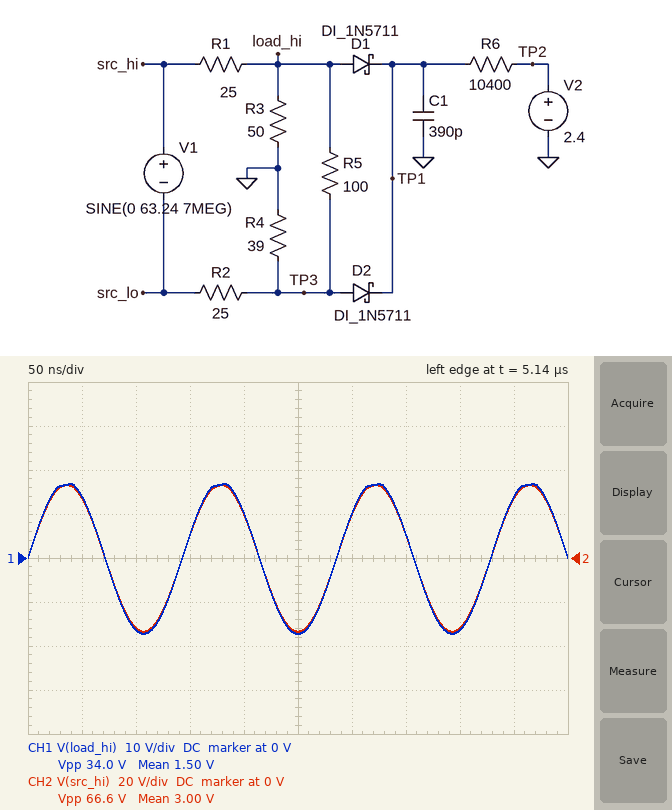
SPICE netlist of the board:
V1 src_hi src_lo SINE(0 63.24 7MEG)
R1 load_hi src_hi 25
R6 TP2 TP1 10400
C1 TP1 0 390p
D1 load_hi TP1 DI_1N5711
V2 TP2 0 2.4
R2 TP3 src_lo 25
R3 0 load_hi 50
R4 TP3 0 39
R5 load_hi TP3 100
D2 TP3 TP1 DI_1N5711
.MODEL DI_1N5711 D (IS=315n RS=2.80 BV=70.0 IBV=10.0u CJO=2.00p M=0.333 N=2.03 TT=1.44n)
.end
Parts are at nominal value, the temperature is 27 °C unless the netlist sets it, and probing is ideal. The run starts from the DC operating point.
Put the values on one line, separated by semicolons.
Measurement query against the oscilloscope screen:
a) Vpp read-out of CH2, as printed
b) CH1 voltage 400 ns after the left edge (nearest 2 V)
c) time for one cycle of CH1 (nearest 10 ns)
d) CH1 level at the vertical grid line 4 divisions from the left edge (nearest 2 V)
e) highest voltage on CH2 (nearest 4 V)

66.6 V; -16 V; 140 ns; 10 V; 32 V
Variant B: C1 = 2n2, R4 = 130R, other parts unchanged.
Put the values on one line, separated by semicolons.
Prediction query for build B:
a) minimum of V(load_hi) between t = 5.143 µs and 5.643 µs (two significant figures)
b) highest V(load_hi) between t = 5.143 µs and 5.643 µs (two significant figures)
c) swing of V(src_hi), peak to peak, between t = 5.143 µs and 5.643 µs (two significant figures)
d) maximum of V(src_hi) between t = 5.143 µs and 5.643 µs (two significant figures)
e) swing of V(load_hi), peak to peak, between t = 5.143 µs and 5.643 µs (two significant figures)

-11 V; 9.9 V; 49 V; 24 V; 21 V
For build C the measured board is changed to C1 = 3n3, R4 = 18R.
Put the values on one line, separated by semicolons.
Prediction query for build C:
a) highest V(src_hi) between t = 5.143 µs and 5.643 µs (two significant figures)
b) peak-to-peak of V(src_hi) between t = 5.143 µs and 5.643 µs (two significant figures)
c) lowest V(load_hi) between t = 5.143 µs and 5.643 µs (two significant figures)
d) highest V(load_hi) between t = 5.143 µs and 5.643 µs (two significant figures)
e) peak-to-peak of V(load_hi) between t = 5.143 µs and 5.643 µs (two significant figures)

38 V; 76 V; -21 V; 20 V; 41 V
